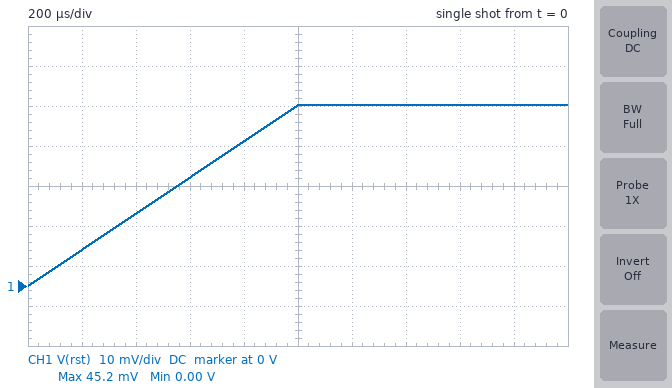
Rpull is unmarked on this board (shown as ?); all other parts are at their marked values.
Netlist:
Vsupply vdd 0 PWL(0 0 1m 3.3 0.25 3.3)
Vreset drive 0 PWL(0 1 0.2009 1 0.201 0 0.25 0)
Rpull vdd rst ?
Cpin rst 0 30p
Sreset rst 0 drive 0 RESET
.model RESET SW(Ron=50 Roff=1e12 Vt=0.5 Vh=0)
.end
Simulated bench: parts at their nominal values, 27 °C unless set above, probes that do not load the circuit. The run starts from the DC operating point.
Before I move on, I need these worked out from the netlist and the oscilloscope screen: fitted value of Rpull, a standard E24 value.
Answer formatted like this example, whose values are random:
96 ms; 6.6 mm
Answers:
3.6 kΩ
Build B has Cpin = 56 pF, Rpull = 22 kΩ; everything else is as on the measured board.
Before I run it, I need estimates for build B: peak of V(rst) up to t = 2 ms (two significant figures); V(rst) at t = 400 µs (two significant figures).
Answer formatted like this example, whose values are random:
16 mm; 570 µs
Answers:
7.5 mV; 3.0 mV
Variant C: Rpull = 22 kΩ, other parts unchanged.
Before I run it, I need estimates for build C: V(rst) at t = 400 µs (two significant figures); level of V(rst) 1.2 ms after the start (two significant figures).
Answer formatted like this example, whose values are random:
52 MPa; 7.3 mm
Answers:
3.0 mV; 7.5 mV
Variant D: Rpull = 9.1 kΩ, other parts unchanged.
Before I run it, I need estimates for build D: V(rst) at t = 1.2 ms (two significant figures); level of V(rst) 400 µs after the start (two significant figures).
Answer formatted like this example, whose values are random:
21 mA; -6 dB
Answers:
18 mV; 7.2 mV
